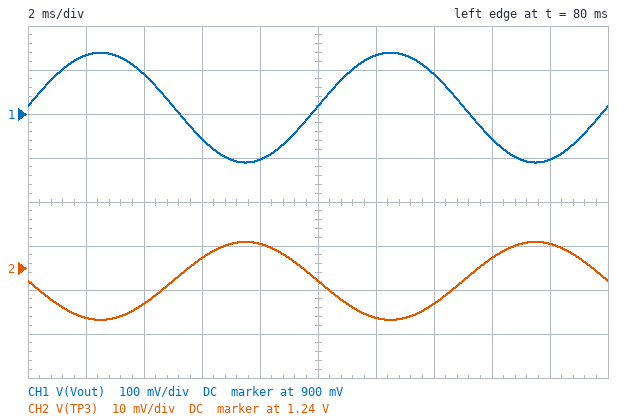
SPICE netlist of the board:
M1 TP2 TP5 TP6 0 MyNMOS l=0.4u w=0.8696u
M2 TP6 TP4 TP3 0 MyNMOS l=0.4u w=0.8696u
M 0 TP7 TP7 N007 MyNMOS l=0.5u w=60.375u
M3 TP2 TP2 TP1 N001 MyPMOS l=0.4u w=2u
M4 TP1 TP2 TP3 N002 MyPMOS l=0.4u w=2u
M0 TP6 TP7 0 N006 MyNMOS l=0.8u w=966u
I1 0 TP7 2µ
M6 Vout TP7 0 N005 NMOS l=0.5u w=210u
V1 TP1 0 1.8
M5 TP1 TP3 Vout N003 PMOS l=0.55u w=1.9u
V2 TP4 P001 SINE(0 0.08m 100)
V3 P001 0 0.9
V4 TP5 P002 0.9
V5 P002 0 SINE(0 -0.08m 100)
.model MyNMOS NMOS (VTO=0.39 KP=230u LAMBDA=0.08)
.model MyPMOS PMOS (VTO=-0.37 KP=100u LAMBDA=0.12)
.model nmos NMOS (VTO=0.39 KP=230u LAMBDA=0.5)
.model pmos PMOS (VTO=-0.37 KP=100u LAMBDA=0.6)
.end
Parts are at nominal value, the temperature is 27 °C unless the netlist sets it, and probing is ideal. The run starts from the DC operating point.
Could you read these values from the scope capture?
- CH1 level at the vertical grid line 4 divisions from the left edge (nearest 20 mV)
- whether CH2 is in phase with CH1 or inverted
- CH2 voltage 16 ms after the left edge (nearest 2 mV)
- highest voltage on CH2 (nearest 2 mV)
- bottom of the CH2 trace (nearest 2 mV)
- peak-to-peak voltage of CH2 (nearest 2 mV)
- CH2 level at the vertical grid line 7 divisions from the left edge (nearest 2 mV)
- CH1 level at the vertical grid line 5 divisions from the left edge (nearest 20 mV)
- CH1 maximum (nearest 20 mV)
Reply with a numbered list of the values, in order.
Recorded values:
1. 800 mV
2. inverted
3. 1.242 V
4. 1.246 V
5. 1.228 V
6. 18 mV
7. 1.232 V
8. 920 mV
9. 1.04 V
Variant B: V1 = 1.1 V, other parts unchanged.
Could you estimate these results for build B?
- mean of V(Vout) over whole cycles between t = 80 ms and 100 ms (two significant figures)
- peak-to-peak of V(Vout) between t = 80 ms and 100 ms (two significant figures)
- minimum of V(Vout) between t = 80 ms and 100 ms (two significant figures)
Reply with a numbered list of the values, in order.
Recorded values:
1. 540 mV
2. 210 mV
3. 440 mV
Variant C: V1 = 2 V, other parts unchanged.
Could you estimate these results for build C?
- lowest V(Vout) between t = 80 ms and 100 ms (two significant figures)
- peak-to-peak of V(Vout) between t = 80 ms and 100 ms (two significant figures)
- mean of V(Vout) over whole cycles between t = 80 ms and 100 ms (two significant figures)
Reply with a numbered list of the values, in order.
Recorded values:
1. 890 mV
2. 260 mV
3. 1.0 V
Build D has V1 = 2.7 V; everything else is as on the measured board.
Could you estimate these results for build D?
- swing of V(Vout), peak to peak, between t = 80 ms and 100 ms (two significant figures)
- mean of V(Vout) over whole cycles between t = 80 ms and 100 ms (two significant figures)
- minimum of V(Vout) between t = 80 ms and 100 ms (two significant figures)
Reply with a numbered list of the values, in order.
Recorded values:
1. 310 mV
2. 1.4 V
3. 1.2 V
